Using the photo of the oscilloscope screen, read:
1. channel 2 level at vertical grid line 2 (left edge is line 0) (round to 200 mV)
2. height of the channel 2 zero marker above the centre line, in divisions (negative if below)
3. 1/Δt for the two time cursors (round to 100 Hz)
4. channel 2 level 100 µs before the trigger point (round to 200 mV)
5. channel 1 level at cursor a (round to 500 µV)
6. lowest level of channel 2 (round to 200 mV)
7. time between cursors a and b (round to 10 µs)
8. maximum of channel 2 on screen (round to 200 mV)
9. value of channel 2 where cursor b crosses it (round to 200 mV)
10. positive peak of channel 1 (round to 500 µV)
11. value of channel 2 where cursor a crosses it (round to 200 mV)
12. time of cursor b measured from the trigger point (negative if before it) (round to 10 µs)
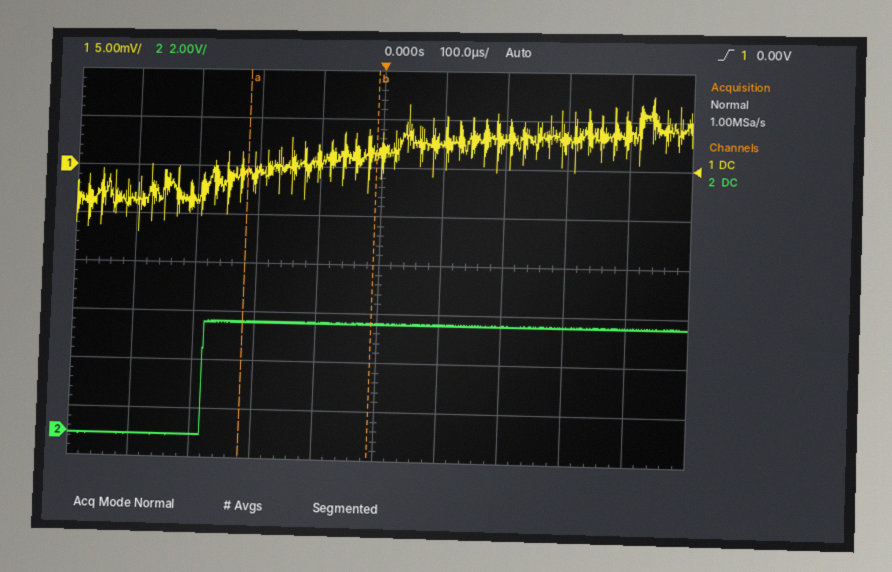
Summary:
0.0 V
-3.5 div
4.8 kHz
4.6 V
-500 µV
0.0 V
210 µs
4.6 V
4.6 V
7.5 mV
4.6 V
-10 µs
